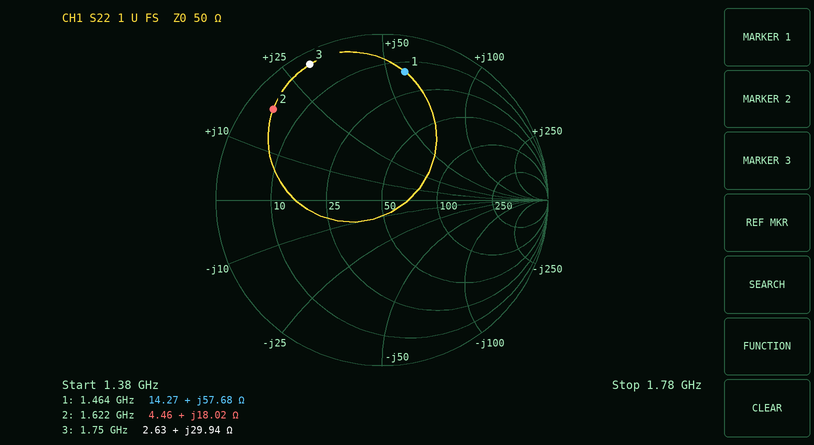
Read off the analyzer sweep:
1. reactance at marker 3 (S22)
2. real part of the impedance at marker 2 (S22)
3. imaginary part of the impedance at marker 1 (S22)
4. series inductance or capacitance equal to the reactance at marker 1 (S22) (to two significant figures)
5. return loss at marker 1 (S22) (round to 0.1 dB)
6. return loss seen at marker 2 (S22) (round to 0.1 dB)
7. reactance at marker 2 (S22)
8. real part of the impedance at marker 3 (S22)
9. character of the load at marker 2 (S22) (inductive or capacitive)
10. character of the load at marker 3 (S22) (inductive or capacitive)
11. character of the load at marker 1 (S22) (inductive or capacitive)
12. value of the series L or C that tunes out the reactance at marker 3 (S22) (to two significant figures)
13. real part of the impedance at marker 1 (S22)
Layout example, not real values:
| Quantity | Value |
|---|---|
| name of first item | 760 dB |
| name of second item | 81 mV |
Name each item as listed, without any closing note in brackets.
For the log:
| Quantity | Value |
|---|---|
| reactance at marker 3 | +29.94 Ω |
| real part of the impedance at marker 2 | 4.46 Ω |
| imaginary part of the impedance at marker 1 | +57.68 Ω |
| series inductance or capacitance equal to the reactance at marker 1 (S22) | 6.3 nH |
| return loss at marker 1 (S22) | 2.1 dB |
| return loss seen at marker 2 (S22) | 1.4 dB |
| reactance at marker 2 | +18.02 Ω |
| real part of the impedance at marker 3 | 2.63 Ω |
| character of the load at marker 2 (S22) | inductive |
| character of the load at marker 3 (S22) | inductive |
| character of the load at marker 1 (S22) | inductive |
| value of the series L or C that tunes out the reactance at marker 3 (S22) | 3.0 pF |
| real part of the impedance at marker 1 | 14.27 Ω |
